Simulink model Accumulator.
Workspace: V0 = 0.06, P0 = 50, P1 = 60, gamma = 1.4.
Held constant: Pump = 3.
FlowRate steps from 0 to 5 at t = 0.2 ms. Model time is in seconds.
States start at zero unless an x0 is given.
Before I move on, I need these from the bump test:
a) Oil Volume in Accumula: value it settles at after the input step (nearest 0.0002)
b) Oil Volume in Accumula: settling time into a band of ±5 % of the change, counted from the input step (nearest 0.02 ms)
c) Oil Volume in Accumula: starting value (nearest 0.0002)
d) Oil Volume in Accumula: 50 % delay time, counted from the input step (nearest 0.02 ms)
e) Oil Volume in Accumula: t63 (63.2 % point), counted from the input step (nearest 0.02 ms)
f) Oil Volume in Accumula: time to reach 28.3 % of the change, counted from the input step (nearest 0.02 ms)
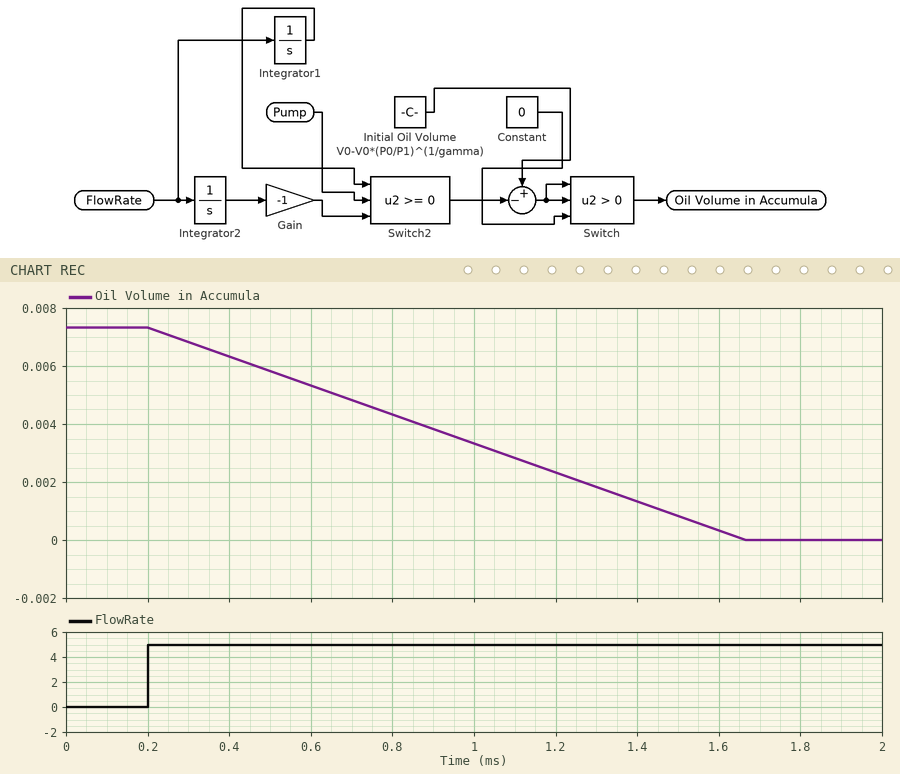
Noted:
0.0000
1.40 ms
0.0074
0.74 ms
0.92 ms
0.42 ms
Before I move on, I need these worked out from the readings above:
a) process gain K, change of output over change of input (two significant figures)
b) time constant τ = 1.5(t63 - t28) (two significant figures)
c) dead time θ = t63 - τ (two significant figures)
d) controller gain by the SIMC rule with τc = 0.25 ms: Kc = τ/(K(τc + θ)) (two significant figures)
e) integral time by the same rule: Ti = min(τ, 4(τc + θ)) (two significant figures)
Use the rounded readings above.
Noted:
-0.0015
0.75 ms
0.17 ms
-1200
0.75 ms
